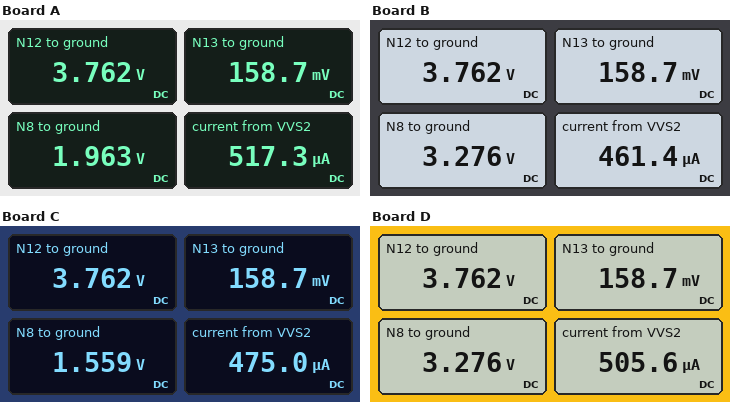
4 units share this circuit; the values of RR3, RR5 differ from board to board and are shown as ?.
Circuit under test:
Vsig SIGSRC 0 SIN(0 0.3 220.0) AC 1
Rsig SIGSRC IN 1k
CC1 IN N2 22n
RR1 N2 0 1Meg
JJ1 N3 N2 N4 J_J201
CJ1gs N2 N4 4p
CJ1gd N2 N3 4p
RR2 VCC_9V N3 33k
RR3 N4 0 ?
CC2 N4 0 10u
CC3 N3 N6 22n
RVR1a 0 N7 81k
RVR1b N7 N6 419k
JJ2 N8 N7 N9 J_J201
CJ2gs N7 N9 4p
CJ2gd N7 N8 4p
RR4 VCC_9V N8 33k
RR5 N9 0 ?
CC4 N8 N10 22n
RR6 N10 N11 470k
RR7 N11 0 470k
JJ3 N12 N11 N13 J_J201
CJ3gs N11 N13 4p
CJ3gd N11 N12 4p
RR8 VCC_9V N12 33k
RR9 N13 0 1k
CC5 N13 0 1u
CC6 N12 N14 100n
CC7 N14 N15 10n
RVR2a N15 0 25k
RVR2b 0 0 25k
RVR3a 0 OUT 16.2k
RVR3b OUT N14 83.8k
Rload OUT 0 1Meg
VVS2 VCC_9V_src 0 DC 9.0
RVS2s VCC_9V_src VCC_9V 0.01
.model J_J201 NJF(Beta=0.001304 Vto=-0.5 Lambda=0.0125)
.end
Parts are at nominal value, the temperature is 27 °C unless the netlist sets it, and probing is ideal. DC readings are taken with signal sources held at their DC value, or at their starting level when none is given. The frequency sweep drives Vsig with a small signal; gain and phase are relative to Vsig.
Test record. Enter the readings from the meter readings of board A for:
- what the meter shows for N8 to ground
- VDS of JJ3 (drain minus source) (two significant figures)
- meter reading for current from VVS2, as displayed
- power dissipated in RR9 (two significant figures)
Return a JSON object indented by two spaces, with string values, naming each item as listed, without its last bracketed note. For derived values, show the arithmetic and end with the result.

{
  "what the meter shows for N8 to ground": "1.963 V",
  "VDS of JJ3 (drain minus source)": "3.762 V - 158.7 mV = 3.6 V",
  "meter reading for current from VVS2, as displayed": "517.3 µA",
  "power dissipated in RR9": "(158.7 mV)^2 / 1 kΩ = 25 µW"
}
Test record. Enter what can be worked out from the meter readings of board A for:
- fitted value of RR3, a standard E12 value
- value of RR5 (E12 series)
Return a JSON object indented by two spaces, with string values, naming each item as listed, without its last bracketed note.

{
  "fitted value of RR3, a standard E12 value": "1.2 kΩ",
  "value of RR5": "470 Ω"
}
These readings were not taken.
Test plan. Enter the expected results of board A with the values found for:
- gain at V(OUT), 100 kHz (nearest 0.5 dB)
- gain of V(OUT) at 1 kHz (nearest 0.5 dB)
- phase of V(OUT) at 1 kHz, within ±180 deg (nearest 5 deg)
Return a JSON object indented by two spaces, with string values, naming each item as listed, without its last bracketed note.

{
  "gain at V(OUT), 100 kHz": "7.5 dB",
  "gain of V(OUT) at 1 kHz": "39.0 dB",
  "phase of V(OUT) at 1 kHz, within ±180 deg": "170 deg"
}
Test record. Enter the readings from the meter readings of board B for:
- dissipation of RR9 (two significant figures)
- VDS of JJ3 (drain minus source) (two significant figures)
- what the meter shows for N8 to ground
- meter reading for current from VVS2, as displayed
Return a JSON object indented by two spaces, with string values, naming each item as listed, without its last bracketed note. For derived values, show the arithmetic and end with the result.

{
  "dissipation of RR9": "(158.7 mV)^2 / 1 kΩ = 25 µW",
  "VDS of JJ3 (drain minus source)": "3.762 V - 158.7 mV = 3.6 V",
  "what the meter shows for N8 to ground": "3.276 V",
  "meter reading for current from VVS2, as displayed": "461.4 µA"
}
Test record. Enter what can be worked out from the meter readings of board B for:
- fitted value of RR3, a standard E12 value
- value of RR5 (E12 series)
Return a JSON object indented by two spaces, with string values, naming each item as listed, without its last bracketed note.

{
  "fitted value of RR3, a standard E12 value": "1.5 kΩ",
  "value of RR5": "820 Ω"
}
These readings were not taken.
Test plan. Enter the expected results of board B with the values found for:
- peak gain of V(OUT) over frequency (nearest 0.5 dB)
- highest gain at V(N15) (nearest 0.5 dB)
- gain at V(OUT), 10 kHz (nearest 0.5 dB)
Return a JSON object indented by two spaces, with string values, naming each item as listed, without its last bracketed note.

{
  "peak gain of V(OUT) over frequency": "37.5 dB",
  "highest gain at V(N15)": "51.0 dB",
  "gain at V(OUT), 10 kHz": "33.0 dB"
}
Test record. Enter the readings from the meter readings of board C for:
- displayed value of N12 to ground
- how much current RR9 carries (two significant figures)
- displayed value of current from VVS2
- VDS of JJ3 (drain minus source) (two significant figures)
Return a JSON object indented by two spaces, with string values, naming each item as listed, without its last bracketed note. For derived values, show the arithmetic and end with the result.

{
  "displayed value of N12 to ground": "3.762 V",
  "how much current RR9 carries": "(158.7 mV) / 1 kΩ = 160 µA",
  "displayed value of current from VVS2": "475.0 µA",
  "VDS of JJ3 (drain minus source)": "3.762 V - 158.7 mV = 3.6 V"
}
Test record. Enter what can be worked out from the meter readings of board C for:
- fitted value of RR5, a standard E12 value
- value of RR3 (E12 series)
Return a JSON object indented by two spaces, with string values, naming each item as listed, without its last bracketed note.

{
  "fitted value of RR5, a standard E12 value": "390 Ω",
  "value of RR3": "2.7 kΩ"
}
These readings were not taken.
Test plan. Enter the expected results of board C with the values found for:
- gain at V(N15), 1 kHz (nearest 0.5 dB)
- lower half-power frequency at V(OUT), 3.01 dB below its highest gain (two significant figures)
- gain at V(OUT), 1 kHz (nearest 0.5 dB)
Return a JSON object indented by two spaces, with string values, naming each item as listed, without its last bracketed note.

{
  "gain at V(N15), 1 kHz": "52.0 dB",
  "lower half-power frequency at V(OUT), 3.01 dB below its highest gain": "47 Hz",
  "gain at V(OUT), 1 kHz": "37.5 dB"
}
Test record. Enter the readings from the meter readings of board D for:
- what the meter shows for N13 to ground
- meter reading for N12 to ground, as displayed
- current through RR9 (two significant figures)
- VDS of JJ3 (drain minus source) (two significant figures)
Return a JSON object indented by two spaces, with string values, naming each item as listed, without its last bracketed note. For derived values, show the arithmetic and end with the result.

{
  "what the meter shows for N13 to ground": "158.7 mV",
  "meter reading for N12 to ground, as displayed": "3.762 V",
  "current through RR9": "(158.7 mV) / 1 kΩ = 160 µA",
  "VDS of JJ3 (drain minus source)": "3.762 V - 158.7 mV = 3.6 V"
}
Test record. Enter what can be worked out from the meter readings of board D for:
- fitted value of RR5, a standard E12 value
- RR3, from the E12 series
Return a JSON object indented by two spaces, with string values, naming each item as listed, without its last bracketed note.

{
  "fitted value of RR5, a standard E12 value": "820 Ω",
  "RR3, from the E12 series": "820 Ω"
}
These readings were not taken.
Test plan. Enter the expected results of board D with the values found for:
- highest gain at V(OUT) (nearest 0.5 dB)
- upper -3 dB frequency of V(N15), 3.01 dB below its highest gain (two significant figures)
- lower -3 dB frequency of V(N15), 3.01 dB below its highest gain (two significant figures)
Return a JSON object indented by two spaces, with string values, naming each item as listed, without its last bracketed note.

{
  "highest gain at V(OUT)": "38.5 dB",
  "upper -3 dB frequency of V(N15), 3.01 dB below its highest gain": "12 kHz",
  "lower -3 dB frequency of V(N15), 3.01 dB below its highest gain": "430 Hz"
}
